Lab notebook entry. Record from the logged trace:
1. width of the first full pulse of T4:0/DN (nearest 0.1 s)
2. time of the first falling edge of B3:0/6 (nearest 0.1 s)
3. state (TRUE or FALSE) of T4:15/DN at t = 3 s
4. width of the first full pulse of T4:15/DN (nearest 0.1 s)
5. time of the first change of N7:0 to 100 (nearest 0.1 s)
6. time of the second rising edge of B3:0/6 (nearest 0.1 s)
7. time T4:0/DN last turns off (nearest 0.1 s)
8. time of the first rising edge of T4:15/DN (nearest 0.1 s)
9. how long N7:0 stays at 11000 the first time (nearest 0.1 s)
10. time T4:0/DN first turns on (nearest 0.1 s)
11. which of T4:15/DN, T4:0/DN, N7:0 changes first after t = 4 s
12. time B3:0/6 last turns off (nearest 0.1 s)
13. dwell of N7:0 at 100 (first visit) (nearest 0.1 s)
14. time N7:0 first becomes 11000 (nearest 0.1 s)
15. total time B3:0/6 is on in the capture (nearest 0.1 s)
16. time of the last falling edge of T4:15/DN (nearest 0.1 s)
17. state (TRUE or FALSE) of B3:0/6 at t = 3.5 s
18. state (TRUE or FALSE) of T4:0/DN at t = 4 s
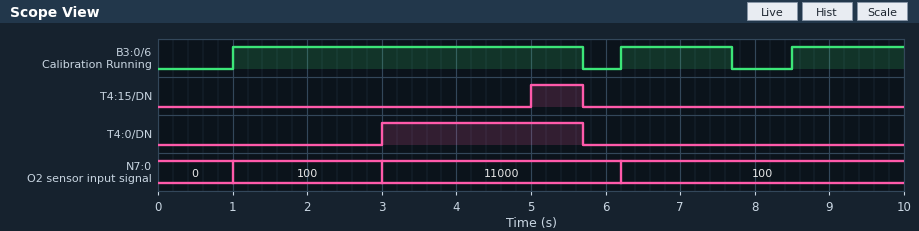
2.7 s
5.7 s
FALSE
0.7 s
1.0 s
6.2 s
5.7 s
5.0 s
3.2 s
3.0 s
T4:15/DN
7.7 s
2.0 s
3.0 s
7.7 s
5.7 s
TRUE
TRUE
